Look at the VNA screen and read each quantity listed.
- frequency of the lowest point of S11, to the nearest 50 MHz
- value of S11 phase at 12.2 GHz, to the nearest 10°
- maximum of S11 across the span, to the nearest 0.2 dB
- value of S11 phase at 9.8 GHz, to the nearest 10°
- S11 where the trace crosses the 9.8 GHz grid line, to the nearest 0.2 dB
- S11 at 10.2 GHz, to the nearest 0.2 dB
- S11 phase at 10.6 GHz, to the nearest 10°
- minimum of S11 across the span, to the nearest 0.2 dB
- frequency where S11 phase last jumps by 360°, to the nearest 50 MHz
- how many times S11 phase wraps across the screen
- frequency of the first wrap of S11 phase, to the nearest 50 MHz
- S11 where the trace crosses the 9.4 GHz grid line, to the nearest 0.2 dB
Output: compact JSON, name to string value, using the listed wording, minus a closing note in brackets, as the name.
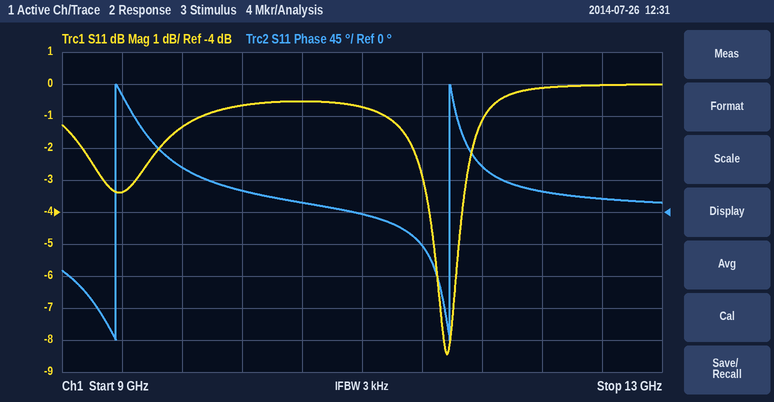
{"frequency of the lowest point of S11, to the nearest 50 MHz": "11.55 GHz", "value of S11 phase at 12.2 GHz, to the nearest 10°": "30°", "maximum of S11 across the span, to the nearest 0.2 dB": "0.0 dB", "value of S11 phase at 9.8 GHz, to the nearest 10°": "60°", "S11 where the trace crosses the 9.8 GHz grid line, to the nearest 0.2 dB": "-1.4 dB", "S11 at 10.2 GHz, to the nearest 0.2 dB": "-0.6 dB", "S11 phase at 10.6 GHz, to the nearest 10°": "10°", "minimum of S11 across the span, to the nearest 0.2 dB": "-8.4 dB", "frequency where S11 phase last jumps by 360°, to the nearest 50 MHz": "11.60 GHz", "how many times S11 phase wraps across the screen": "2", "frequency of the first wrap of S11 phase, to the nearest 50 MHz": "9.35 GHz", "S11 where the trace crosses the 9.4 GHz grid line, to the nearest 0.2 dB": "-3.4 dB"}
